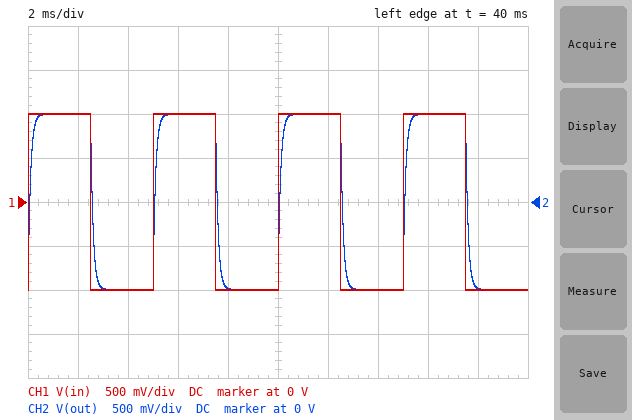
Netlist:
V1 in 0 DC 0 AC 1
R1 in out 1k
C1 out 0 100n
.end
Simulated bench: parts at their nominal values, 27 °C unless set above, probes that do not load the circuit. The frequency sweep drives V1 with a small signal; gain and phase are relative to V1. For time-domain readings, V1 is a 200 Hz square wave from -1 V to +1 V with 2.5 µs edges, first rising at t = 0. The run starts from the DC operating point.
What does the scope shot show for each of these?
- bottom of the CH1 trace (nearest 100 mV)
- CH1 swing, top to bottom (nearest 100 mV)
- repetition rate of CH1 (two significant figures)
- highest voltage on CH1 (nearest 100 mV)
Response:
-1.0 V
2.0 V
200 Hz
1.0 V
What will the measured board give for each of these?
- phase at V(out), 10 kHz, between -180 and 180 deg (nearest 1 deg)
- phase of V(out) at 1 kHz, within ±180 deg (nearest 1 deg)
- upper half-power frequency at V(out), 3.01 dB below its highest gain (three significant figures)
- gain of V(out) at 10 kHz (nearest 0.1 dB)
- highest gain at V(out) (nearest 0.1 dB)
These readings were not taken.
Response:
-81 deg
-32 deg
1.59 kHz
-16.1 dB
0 dB
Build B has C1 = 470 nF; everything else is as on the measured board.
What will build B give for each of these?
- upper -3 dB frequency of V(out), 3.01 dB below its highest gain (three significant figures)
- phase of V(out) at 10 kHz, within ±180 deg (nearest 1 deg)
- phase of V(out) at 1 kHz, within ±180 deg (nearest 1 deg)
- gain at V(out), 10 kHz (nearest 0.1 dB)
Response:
339 Hz
-88 deg
-71 deg
-29.4 dB
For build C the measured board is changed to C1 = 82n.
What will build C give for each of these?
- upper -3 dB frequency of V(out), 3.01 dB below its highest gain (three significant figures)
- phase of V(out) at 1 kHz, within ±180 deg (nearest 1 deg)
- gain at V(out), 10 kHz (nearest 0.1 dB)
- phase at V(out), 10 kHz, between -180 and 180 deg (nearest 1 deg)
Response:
1.94 kHz
-27 deg
-14.4 dB
-79 deg
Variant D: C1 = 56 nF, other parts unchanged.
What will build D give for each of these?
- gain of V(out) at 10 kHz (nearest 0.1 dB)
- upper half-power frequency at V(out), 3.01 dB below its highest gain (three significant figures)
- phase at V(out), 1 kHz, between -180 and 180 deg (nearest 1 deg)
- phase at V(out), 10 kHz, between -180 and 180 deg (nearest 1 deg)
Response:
-11.3 dB
2.84 kHz
-19 deg
-74 deg
